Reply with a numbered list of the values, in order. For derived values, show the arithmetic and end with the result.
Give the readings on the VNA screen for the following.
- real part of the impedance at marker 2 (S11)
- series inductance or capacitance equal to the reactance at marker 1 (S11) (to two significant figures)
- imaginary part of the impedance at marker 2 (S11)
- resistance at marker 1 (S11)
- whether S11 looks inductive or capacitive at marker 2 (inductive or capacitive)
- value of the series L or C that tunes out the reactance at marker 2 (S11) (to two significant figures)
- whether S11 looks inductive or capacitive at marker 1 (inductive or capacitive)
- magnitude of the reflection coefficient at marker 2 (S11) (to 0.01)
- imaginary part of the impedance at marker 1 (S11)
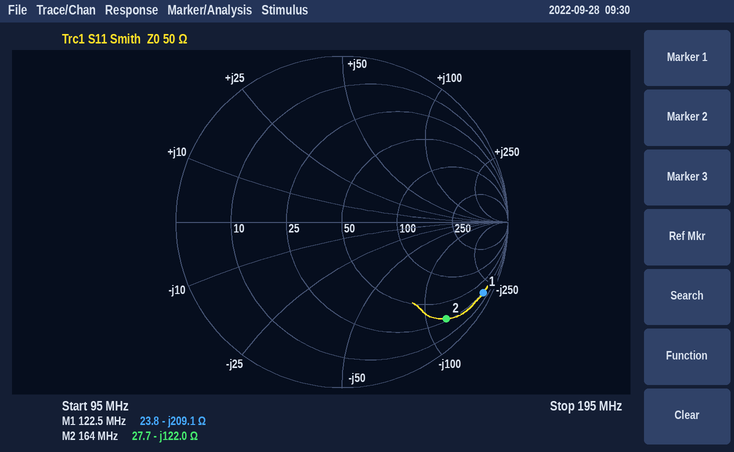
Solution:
1. 27.7 Ω
2. C = 1/(2π × 122.5 MHz × 209.1 Ω) ≈ 6.2 pF
3. -122.0 Ω
4. 23.8 Ω
5. capacitive
6. L = 122 Ω/(2π × 164 MHz) ≈ 118 nH, so 120 nH to two significant figures
7. capacitive
8. 0.86
9. -209.1 Ω
